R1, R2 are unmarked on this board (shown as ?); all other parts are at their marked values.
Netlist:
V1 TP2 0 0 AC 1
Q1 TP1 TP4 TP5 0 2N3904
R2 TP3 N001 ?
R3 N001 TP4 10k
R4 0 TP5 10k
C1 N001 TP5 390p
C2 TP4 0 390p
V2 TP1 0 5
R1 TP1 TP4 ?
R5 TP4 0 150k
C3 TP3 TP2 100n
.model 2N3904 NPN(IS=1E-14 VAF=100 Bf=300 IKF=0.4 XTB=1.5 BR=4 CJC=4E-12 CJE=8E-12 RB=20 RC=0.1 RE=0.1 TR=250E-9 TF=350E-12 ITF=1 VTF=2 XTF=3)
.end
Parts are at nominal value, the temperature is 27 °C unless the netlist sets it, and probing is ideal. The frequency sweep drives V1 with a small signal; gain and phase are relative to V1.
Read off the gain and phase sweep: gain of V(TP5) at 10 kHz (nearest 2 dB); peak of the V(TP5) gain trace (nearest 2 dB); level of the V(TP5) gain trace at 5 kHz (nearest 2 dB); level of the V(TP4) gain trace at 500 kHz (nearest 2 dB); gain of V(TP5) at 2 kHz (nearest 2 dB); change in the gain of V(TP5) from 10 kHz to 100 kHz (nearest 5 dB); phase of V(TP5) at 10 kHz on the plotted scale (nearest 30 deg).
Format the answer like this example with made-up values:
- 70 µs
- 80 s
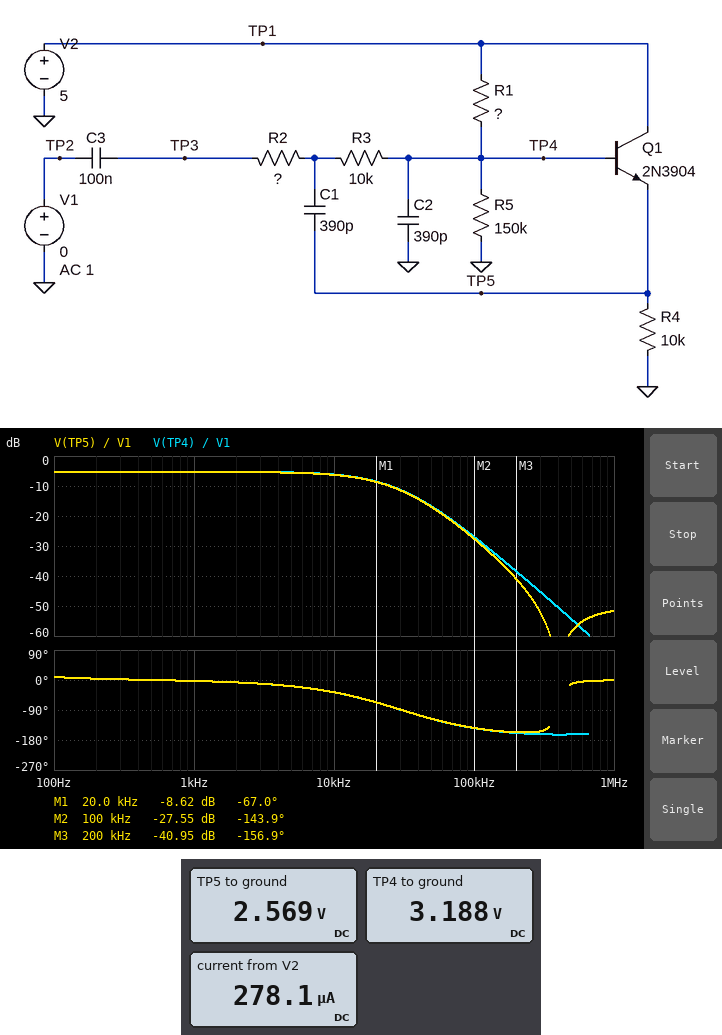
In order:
- -6 dB
- -6 dB
- -6 dB
- -54 dB
- -6 dB
- -20 dB
- -30 deg
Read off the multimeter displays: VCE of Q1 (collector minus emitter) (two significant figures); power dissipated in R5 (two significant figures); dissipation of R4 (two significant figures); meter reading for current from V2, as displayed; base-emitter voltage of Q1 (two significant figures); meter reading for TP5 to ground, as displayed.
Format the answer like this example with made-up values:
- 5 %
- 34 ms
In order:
- 2.4 V
- 68 µW
- 660 µW
- 278.1 µA
- 620 mV
- 2.569 V
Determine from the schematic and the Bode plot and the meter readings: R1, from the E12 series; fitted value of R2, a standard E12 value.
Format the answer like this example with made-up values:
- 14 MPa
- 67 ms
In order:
- 82 kΩ
- 33 kΩ
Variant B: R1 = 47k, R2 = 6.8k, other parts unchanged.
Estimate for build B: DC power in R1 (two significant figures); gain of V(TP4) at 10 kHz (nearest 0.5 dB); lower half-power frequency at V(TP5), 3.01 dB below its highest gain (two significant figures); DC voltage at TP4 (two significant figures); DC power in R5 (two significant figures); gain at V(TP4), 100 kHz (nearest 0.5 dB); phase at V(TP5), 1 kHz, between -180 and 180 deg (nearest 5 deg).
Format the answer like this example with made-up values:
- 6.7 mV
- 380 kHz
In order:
- 32 µW
- -3.5 dB
- 30 Hz
- 3.8 V
- 95 µW
- -14.5 dB
- 0 deg
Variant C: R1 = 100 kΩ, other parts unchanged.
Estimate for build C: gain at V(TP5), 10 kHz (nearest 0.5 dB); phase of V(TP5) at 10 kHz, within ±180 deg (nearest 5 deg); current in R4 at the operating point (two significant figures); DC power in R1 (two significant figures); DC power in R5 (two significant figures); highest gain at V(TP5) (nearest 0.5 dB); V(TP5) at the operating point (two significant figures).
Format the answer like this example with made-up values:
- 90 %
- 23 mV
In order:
- -6.0 dB
- -40 deg
- 230 µA
- 42 µW
- 58 µW
- -5.0 dB
- 2.3 V
